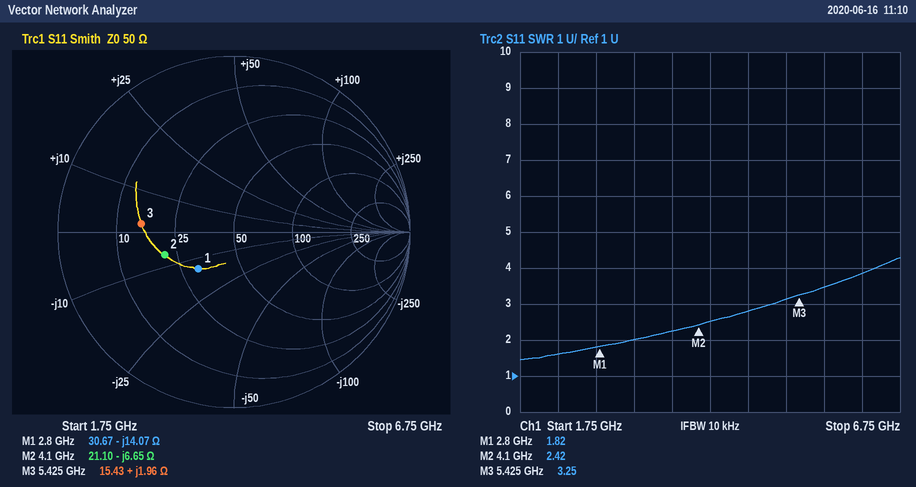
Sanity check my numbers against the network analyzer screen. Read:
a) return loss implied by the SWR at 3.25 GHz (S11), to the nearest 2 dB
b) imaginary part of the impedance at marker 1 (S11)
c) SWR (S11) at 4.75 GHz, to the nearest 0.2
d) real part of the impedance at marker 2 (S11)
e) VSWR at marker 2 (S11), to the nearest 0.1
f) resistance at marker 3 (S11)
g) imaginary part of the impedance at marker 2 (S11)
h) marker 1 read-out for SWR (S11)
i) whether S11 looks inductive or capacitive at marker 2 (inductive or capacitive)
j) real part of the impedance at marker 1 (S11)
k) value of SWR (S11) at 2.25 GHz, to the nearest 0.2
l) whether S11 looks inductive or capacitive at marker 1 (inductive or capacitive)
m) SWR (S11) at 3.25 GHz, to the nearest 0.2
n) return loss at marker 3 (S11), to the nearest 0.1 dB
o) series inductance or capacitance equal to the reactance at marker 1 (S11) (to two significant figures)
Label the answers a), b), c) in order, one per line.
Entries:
a) 10 dB
b) -14.07 Ω
c) 2.8
d) 21.10 Ω
e) 2.4
f) 15.43 Ω
g) -6.65 Ω
h) 1.82
i) capacitive
j) 30.67 Ω
k) 1.6
l) capacitive
m) 2.0
n) 5.5 dB
o) 4.0 pF
